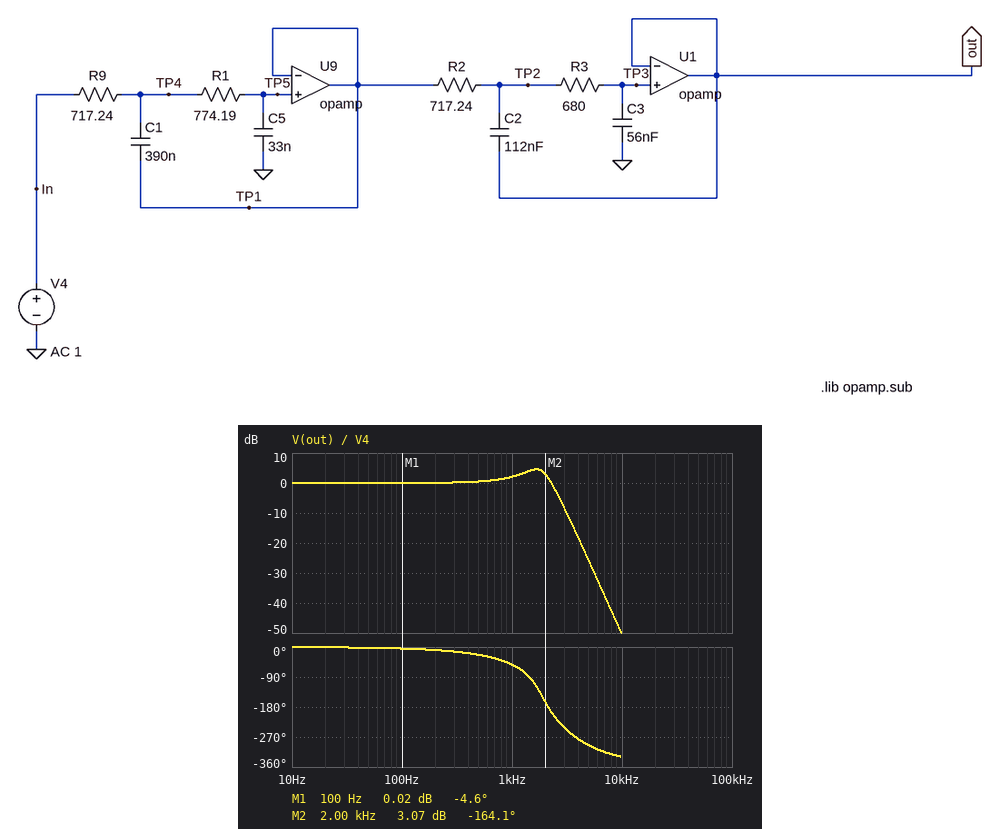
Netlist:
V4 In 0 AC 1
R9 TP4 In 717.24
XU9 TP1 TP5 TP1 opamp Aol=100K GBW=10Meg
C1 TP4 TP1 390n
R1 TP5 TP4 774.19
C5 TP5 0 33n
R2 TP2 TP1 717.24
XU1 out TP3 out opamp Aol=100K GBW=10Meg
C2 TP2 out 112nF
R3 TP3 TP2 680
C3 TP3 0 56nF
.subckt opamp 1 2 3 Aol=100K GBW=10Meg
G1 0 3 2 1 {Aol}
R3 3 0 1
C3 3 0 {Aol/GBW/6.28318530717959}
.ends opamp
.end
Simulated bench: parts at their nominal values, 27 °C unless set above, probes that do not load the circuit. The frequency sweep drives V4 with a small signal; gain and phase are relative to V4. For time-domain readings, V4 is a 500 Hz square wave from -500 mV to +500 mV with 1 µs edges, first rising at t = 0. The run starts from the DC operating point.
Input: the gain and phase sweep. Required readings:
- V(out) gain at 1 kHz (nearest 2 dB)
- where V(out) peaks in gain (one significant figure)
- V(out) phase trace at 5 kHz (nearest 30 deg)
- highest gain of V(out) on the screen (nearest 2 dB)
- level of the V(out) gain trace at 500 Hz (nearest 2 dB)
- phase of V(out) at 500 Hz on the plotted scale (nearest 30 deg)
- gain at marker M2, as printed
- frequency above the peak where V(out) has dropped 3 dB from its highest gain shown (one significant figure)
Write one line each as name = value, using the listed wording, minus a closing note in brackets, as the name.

V(out) gain at 1 kHz = 2 dB
where V(out) peaks in gain = 2 kHz
V(out) phase trace at 5 kHz = -300 deg
highest gain of V(out) on the screen = 4 dB
level of the V(out) gain trace at 500 Hz = 0 dB
phase of V(out) at 500 Hz on the plotted scale = -30 deg
gain at marker M2, as printed = 3.07 dB
frequency above the peak where V(out) has dropped 3 dB from its highest gain shown = 2 kHz
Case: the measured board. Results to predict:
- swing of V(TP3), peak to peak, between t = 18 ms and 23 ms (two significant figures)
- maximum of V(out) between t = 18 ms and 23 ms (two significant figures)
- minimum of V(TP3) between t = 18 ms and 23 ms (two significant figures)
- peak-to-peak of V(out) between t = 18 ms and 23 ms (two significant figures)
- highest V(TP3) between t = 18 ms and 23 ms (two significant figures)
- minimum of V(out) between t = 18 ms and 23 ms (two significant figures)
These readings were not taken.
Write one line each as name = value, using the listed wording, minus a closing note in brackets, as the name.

swing of V(TP3), peak to peak, between t = 18 ms and 23 ms = 1.7 V
maximum of V(out) between t = 18 ms and 23 ms = 870 mV
minimum of V(TP3) between t = 18 ms and 23 ms = -870 mV
peak-to-peak of V(out) between t = 18 ms and 23 ms = 1.7 V
highest V(TP3) between t = 18 ms and 23 ms = 870 mV
minimum of V(out) between t = 18 ms and 23 ms = -870 mV
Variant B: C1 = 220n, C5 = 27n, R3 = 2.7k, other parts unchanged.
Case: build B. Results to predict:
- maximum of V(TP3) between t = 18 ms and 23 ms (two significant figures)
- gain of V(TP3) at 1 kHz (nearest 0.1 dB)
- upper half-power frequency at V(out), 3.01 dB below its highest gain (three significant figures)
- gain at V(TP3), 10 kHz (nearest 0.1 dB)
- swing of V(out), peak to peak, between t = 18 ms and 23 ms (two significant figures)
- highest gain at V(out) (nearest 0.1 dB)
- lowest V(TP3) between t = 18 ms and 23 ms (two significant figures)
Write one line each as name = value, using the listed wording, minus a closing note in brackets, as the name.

maximum of V(TP3) between t = 18 ms and 23 ms = 510 mV
gain of V(TP3) at 1 kHz = -1.5 dB
upper half-power frequency at V(out), 3.01 dB below its highest gain = 1.44 kHz
gain at V(TP3), 10 kHz = -55.5 dB
swing of V(out), peak to peak, between t = 18 ms and 23 ms = 1.0 V
highest gain at V(out) = 0 dB
lowest V(TP3) between t = 18 ms and 23 ms = -510 mV
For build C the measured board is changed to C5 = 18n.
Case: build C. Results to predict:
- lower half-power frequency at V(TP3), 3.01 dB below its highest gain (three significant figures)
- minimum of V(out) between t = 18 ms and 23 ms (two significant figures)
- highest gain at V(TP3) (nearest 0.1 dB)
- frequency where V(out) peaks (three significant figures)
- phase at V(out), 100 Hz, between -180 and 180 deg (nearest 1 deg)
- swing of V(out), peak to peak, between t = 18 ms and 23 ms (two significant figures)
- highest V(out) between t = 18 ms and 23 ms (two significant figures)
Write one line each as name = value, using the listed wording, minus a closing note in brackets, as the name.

lower half-power frequency at V(TP3), 3.01 dB below its highest gain = 1.52 kHz
minimum of V(out) between t = 18 ms and 23 ms = -930 mV
highest gain at V(TP3) = 5.9 dB
frequency where V(out) peaks = 2.34 kHz
phase at V(out), 100 Hz, between -180 and 180 deg = -4 deg
swing of V(out), peak to peak, between t = 18 ms and 23 ms = 1.9 V
highest V(out) between t = 18 ms and 23 ms = 930 mV
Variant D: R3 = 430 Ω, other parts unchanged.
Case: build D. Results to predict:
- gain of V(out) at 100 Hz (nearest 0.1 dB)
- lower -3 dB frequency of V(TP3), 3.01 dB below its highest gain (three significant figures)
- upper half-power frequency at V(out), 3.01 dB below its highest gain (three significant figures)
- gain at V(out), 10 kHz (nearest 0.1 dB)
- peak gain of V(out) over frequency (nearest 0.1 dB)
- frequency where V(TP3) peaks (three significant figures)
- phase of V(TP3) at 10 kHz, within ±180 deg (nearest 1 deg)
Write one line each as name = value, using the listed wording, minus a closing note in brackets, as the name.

gain of V(out) at 100 Hz = 0 dB
lower -3 dB frequency of V(TP3), 3.01 dB below its highest gain = 919 Hz
upper half-power frequency at V(out), 3.01 dB below its highest gain = 2.18 kHz
gain at V(out), 10 kHz = -46.6 dB
peak gain of V(out) over frequency = 4.8 dB
frequency where V(TP3) peaks = 1.69 kHz
phase of V(TP3) at 10 kHz, within ±180 deg = 38 deg
